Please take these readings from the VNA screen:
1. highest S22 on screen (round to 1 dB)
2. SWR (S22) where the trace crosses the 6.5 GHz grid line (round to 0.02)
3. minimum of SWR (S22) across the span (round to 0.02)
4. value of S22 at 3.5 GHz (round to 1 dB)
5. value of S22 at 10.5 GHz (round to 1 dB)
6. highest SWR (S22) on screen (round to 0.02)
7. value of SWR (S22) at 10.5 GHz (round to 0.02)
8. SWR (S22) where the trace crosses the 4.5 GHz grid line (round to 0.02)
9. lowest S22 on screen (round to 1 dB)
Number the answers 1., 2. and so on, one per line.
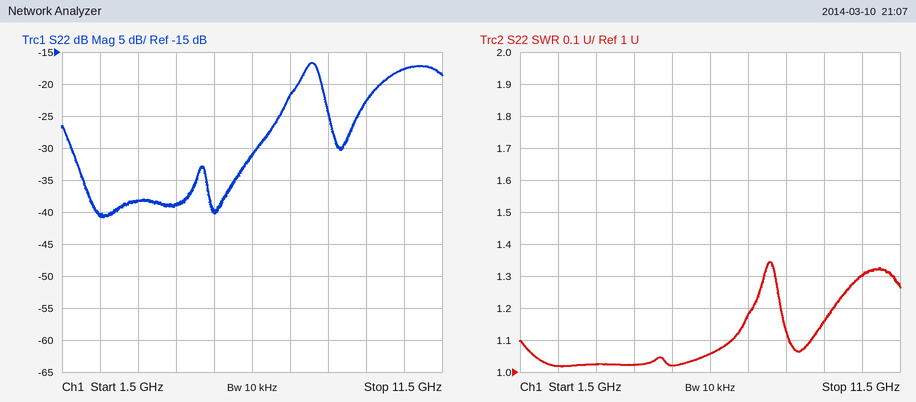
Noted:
1. -17 dB
2. 1.06
3. 1.02
4. -38 dB
5. -18 dB
6. 1.34
7. 1.30
8. 1.02
9. -41 dB
